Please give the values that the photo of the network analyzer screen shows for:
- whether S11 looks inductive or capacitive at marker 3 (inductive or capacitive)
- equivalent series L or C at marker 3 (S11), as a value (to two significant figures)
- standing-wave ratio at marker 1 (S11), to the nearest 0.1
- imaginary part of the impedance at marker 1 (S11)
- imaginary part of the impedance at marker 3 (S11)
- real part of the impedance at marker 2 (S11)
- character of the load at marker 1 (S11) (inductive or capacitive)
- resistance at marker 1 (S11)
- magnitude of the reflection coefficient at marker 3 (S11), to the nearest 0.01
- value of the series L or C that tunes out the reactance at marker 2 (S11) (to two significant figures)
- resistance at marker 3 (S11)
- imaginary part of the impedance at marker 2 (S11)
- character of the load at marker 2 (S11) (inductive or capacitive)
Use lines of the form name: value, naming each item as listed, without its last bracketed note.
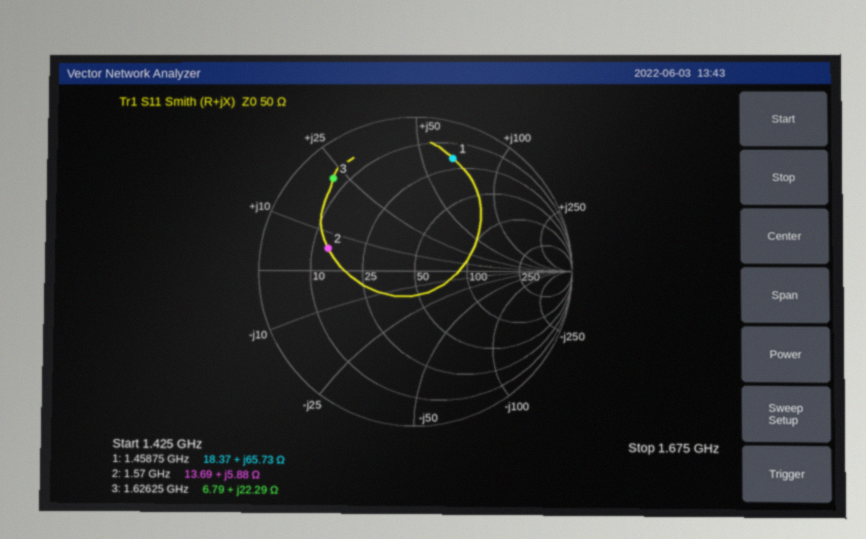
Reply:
whether S11 looks inductive or capacitive at marker 3: inductive
equivalent series L or C at marker 3 (S11), as a value: 2.2 nH
standing-wave ratio at marker 1 (S11), to the nearest 0.1: 7.7
imaginary part of the impedance at marker 1: +65.73 Ω
imaginary part of the impedance at marker 3: +22.29 Ω
real part of the impedance at marker 2: 13.69 Ω
character of the load at marker 1 (S11): inductive
resistance at marker 1: 18.37 Ω
magnitude of the reflection coefficient at marker 3 (S11), to the nearest 0.01: 0.80
value of the series L or C that tunes out the reactance at marker 2 (S11): 17 pF
resistance at marker 3: 6.79 Ω
imaginary part of the impedance at marker 2: +5.88 Ω
character of the load at marker 2 (S11): inductive
